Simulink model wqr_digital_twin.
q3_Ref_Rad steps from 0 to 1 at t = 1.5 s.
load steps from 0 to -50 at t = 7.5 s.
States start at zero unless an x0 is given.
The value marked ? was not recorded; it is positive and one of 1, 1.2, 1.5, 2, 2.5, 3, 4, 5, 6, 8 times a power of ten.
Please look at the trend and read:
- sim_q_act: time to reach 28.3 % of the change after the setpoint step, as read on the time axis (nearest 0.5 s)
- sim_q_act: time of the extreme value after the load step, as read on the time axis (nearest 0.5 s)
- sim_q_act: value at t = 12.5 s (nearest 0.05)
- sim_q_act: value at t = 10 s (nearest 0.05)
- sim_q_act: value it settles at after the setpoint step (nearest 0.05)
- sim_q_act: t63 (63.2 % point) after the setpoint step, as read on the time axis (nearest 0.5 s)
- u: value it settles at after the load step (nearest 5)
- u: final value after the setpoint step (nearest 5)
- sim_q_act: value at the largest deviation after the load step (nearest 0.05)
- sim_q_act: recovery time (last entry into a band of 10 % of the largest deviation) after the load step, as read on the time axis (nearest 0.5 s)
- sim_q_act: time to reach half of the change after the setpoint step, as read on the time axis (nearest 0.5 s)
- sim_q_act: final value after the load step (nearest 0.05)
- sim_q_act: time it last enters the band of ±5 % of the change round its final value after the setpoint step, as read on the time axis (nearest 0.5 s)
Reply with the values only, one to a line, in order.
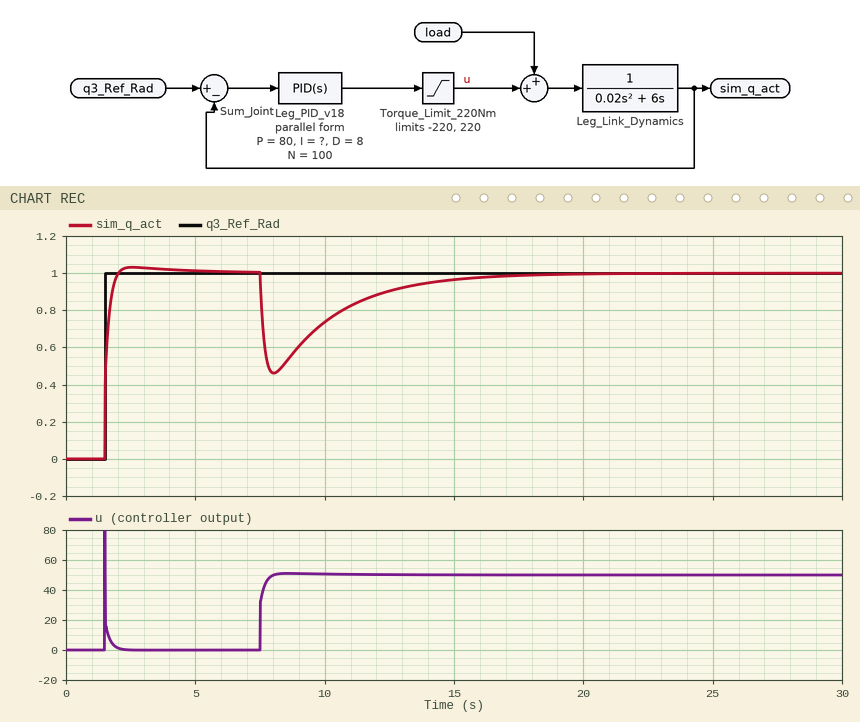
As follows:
1.5 s
8.0 s
0.90
0.75
1.00
1.5 s
50
0
0.45
14.0 s
1.5 s
1.00
2.0 s
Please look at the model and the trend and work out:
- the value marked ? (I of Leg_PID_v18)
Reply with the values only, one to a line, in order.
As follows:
30
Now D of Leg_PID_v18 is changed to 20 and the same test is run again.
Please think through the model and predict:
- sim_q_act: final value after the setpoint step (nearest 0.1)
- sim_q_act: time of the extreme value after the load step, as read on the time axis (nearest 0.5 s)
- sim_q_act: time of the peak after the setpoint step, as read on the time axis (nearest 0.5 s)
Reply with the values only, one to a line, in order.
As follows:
1.0
8.5 s
3.0 s
